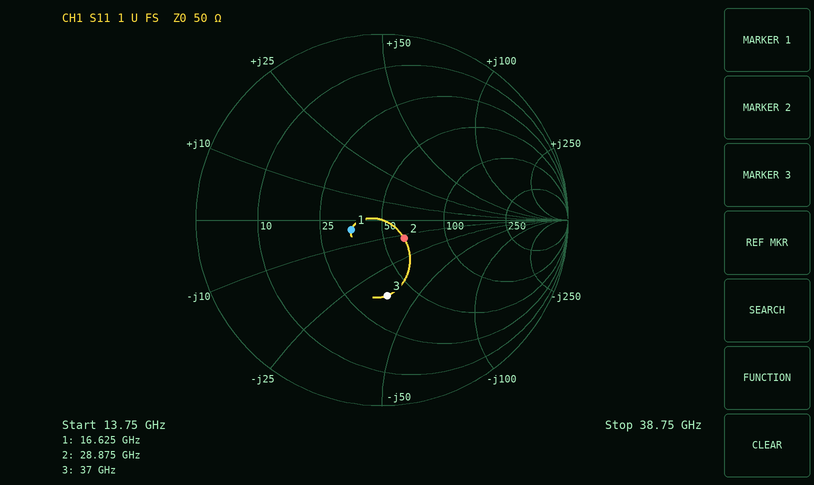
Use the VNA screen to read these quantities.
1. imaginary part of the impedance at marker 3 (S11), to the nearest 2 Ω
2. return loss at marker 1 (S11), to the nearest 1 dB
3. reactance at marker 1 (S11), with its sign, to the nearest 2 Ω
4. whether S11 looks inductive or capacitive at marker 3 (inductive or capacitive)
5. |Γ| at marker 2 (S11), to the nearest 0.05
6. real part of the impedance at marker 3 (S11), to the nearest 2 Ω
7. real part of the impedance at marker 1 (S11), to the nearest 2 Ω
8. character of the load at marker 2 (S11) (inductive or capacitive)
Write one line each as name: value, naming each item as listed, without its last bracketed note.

imaginary part of the impedance at marker 3 (S11), to the nearest 2 Ω: -36 Ω
return loss at marker 1 (S11), to the nearest 1 dB: 15 dB
reactance at marker 1 (S11), with its sign, to the nearest 2 Ω: -4 Ω
whether S11 looks inductive or capacitive at marker 3: capacitive
|Γ| at marker 2 (S11), to the nearest 0.05: 0.15
real part of the impedance at marker 3 (S11), to the nearest 2 Ω: 38 Ω
real part of the impedance at marker 1 (S11), to the nearest 2 Ω: 36 Ω
character of the load at marker 2 (S11): capacitive
